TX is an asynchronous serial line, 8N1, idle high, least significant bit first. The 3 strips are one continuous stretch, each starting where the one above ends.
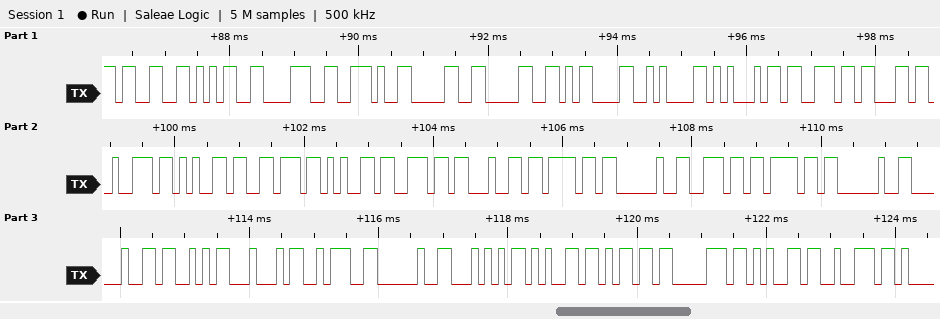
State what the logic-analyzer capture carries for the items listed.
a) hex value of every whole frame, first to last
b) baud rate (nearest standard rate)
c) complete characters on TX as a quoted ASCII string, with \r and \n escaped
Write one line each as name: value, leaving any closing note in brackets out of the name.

hex value of every whole frame, first to last: 33 35 38 2E 30 30 0D 0A 45 73 63 72 65 76 65 6E 64 6F 20 6E 6F 20 20 53 44 3A 20 54 65 6D 70 65 72
baud rate: 9600 baud
complete characters on TX as a quoted ASCII string, with \r and \n escaped: "358.00\r\nEscrevendo no  SD: Temper"
